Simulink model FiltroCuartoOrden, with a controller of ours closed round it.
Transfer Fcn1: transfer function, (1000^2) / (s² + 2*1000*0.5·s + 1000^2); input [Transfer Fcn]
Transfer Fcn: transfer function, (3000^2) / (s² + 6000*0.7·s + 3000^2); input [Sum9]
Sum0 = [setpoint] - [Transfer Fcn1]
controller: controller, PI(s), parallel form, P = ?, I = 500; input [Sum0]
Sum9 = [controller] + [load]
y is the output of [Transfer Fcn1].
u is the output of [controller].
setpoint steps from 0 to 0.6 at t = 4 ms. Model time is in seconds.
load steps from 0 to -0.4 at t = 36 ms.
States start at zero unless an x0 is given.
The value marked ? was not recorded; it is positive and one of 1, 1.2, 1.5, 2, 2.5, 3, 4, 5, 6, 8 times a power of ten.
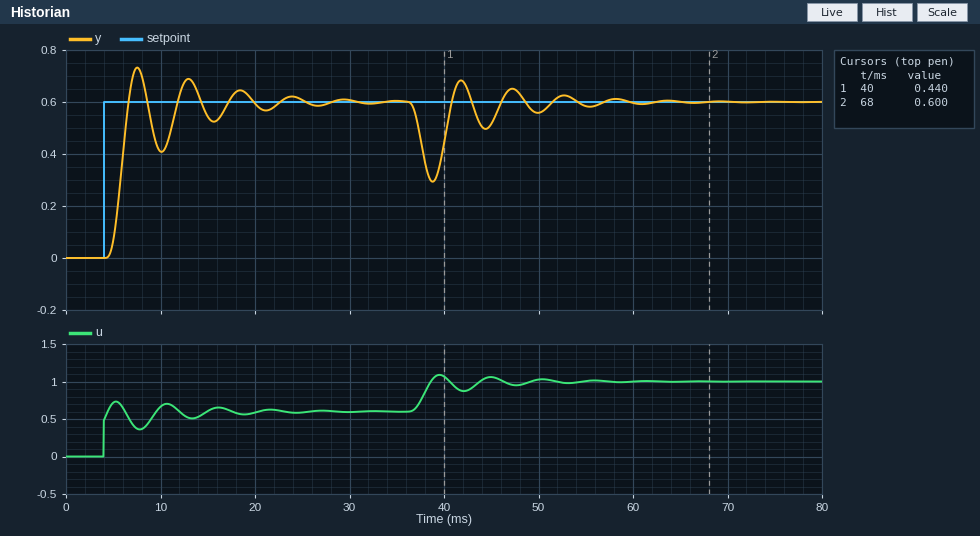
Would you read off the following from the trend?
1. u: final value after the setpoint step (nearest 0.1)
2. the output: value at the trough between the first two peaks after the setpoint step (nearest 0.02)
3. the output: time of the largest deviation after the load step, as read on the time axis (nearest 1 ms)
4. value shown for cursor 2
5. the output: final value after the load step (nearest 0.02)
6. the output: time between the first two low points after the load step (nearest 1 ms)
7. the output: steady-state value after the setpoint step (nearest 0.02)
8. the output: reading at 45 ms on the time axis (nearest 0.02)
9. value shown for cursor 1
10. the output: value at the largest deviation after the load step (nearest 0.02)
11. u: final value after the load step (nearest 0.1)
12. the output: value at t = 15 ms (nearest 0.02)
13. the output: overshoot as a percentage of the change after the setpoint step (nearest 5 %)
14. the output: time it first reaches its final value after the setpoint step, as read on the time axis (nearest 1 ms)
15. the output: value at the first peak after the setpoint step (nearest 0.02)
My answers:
0.6
0.40
39 ms
0.600
0.60
6 ms
0.60
0.52
0.440
0.30
1.0
0.54
20 %
7 ms
0.74
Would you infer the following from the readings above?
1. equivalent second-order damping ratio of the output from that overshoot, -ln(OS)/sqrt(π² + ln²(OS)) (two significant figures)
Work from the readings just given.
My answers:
0.46
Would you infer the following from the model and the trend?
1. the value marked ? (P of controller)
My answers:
0.8
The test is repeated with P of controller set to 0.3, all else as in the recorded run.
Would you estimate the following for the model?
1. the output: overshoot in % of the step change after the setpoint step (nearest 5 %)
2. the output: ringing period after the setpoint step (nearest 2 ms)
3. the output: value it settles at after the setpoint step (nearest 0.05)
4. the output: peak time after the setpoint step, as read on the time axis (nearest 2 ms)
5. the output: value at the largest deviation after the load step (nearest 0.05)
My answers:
25 %
6 ms
0.60
8 ms
0.25
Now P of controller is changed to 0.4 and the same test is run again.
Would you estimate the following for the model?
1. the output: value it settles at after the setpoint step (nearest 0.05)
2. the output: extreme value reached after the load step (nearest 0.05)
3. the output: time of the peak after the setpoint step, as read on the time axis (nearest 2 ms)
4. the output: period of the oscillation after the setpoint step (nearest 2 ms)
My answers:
0.60
0.25
8 ms
6 ms
